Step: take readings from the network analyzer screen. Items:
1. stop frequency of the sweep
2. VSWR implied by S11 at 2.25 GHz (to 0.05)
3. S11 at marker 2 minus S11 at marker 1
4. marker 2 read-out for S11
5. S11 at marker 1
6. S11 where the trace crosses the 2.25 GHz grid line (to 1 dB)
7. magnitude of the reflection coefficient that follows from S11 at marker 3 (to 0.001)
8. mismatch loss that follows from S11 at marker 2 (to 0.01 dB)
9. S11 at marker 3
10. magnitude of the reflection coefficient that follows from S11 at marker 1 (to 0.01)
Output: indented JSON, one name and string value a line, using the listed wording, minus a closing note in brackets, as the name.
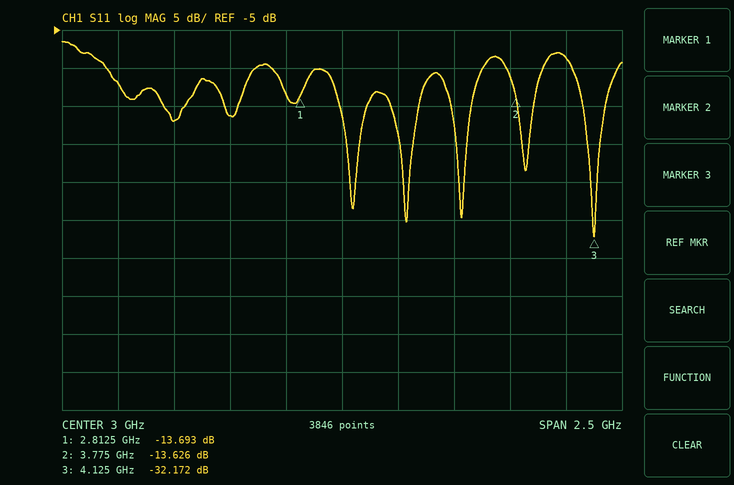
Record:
{
  "stop frequency of the sweep": "4.25 GHz",
  "VSWR implied by S11 at 2.25 GHz": "1.35",
  "S11 at marker 2 minus S11 at marker 1": "0.067 dB",
  "marker 2 read-out for S11": "-13.626 dB",
  "S11 at marker 1": "-13.693 dB",
  "S11 where the trace crosses the 2.25 GHz grid line": "-17 dB",
  "magnitude of the reflection coefficient that follows from S11 at marker 3": "0.025",
  "mismatch loss that follows from S11 at marker 2": "0.19 dB",
  "S11 at marker 3": "-32.172 dB",
  "magnitude of the reflection coefficient that follows from S11 at marker 1": "0.21"
}
